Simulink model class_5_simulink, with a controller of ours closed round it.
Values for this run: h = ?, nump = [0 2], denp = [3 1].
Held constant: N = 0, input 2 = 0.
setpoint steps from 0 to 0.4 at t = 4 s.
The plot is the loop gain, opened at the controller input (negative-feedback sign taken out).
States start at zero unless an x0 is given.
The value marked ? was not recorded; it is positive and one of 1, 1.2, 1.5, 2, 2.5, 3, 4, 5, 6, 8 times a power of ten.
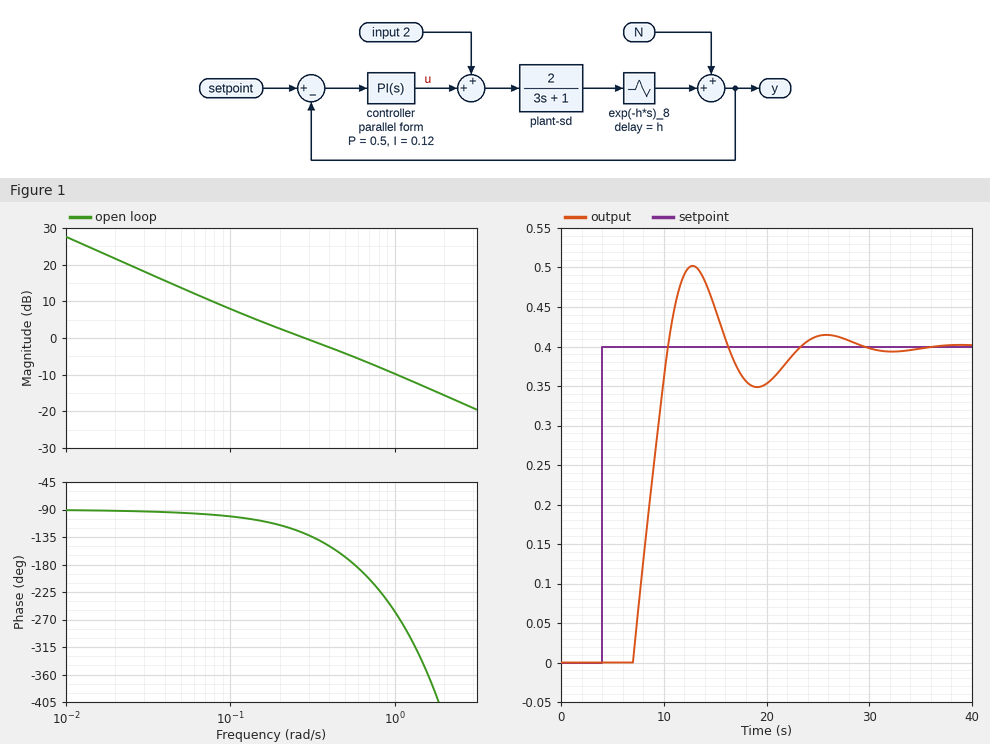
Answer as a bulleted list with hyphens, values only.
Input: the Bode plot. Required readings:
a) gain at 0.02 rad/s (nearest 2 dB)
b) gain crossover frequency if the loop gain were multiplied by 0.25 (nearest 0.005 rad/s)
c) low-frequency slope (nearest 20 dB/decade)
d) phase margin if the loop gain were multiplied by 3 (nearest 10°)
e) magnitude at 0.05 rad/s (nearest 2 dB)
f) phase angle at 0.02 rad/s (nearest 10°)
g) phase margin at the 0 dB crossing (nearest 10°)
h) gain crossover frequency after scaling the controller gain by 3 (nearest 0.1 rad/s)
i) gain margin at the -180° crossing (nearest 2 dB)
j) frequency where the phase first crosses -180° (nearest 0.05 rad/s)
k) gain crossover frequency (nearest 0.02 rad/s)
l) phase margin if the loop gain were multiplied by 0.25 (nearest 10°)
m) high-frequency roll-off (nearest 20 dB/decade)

- 22 dB
- 0.060 rad/s
- -20 dB/decade
- -70°
- 14 dB
- -90°
- 50°
- 1.0 rad/s
- 6 dB
- 0.55 rad/s
- 0.28 rad/s
- 80°
- -20 dB/decade
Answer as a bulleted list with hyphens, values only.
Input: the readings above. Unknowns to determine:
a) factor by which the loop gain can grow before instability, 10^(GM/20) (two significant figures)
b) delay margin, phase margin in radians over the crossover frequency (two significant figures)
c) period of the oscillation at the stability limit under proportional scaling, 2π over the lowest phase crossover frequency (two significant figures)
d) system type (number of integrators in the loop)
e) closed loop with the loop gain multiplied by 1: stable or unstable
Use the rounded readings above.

- 2.0
- 3.1 s
- 11 s
- 1
- stable
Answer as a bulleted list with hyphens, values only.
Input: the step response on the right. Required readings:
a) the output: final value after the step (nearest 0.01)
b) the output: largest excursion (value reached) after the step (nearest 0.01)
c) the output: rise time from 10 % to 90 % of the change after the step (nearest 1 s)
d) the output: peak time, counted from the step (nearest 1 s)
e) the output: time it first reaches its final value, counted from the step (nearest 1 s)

- 0.40
- 0.50
- 3 s
- 9 s
- 6 s
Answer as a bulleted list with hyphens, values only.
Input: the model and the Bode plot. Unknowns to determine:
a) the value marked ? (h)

- 3
